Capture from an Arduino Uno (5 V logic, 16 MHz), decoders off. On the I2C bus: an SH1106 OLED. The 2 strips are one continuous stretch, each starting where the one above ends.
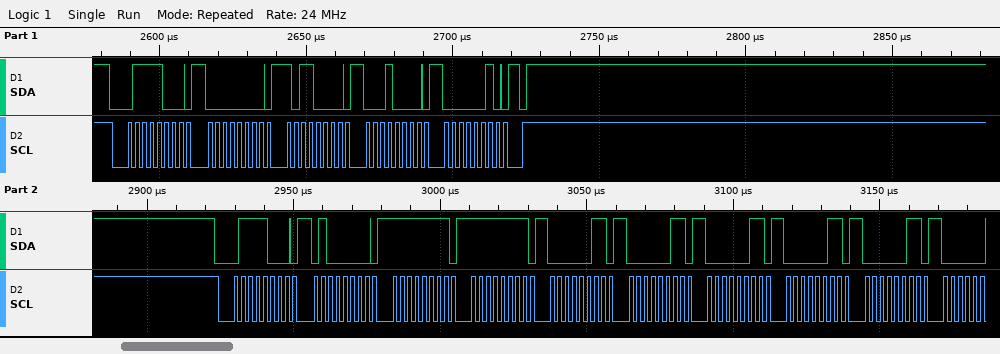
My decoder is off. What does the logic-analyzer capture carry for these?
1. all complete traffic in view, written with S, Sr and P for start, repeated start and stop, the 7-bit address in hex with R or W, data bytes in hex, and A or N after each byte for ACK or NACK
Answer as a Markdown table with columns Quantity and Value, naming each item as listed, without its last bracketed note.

| Quantity | Value |
|---|---|
| all complete traffic in view, written with S, Sr and P for start, repeated start and stop, the 7-bit address in hex with R or W, data bytes in hex, and A or N after each byte for ACK or NACK | S 3CW A 00 A B0 A 10 A 02 A P S 3CW A 40 A FF A FF A 03 A 03 A 03 A 03 A 03 A |
